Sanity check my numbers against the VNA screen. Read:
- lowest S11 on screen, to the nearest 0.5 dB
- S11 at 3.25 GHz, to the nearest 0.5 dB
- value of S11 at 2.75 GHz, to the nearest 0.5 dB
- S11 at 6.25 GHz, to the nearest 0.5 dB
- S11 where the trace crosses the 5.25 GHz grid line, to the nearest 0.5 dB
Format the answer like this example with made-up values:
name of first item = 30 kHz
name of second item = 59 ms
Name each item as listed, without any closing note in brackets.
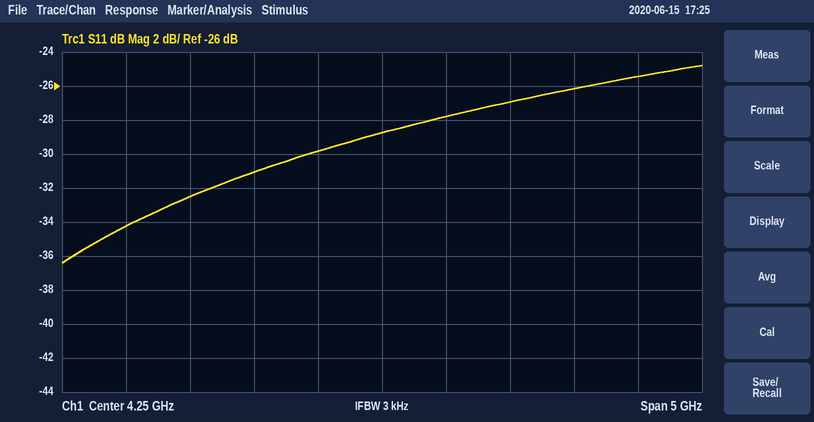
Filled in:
lowest S11 on screen, to the nearest 0.5 dB = -36.5 dB
S11 at 3.25 GHz, to the nearest 0.5 dB = -31.0 dB
value of S11 at 2.75 GHz, to the nearest 0.5 dB = -32.5 dB
S11 at 6.25 GHz, to the nearest 0.5 dB = -25.5 dB
S11 where the trace crosses the 5.25 GHz grid line, to the nearest 0.5 dB = -27.0 dB
